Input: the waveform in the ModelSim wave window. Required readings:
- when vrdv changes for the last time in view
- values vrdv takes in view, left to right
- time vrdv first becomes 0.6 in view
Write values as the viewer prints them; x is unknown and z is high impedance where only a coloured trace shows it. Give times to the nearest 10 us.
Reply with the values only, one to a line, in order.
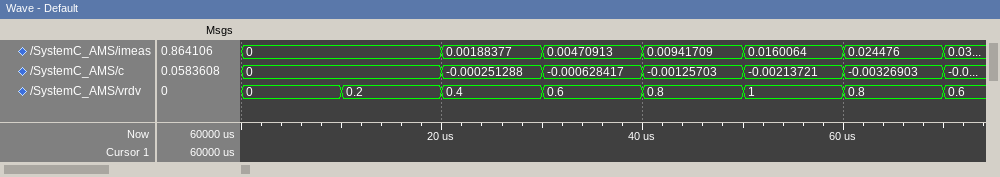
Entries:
70 us
0, 0.2, 0.4, 0.6, 0.8, 1, 0.8, 0.6
30 us
